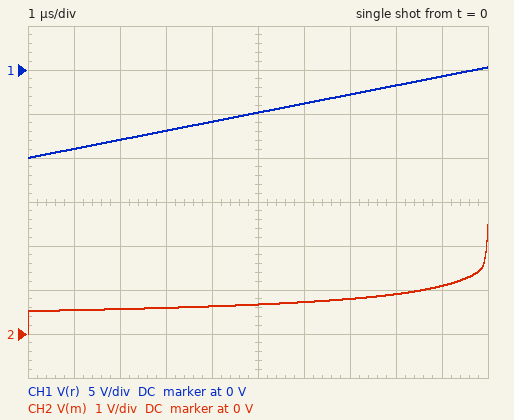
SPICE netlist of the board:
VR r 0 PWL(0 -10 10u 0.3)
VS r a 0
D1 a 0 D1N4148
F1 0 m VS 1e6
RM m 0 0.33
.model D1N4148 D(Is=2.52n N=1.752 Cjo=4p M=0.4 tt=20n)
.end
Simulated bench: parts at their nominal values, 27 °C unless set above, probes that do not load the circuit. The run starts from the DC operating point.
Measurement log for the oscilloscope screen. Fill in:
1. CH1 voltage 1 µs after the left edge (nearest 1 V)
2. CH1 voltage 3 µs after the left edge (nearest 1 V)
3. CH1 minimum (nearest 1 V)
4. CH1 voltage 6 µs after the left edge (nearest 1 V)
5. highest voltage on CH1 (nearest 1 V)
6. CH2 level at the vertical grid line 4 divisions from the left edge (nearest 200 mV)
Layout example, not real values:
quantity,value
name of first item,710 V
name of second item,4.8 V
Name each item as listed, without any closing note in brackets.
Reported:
quantity,value
CH1 voltage 1 µs after the left edge,-9 V
CH1 voltage 3 µs after the left edge,-7 V
CH1 minimum,-10 V
CH1 voltage 6 µs after the left edge,-4 V
highest voltage on CH1,0 V
CH2 level at the vertical grid line 4 divisions from the left edge,600 mV
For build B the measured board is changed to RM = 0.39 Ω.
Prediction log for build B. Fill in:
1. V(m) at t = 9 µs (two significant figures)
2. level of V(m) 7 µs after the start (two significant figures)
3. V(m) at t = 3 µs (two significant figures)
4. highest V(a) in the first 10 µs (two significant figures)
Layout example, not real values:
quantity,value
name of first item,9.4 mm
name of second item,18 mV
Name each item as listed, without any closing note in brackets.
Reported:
quantity,value
V(m) at t = 9 µs,1.3 V
level of V(m) 7 µs after the start,940 mV
V(m) at t = 3 µs,700 mV
highest V(a) in the first 10 µs,300 mV
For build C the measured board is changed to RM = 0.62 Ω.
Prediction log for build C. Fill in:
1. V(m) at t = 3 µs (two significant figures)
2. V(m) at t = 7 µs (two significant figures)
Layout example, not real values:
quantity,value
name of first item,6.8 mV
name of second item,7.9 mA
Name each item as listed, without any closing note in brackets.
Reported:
quantity,value
V(m) at t = 3 µs,1.1 V
V(m) at t = 7 µs,1.5 V
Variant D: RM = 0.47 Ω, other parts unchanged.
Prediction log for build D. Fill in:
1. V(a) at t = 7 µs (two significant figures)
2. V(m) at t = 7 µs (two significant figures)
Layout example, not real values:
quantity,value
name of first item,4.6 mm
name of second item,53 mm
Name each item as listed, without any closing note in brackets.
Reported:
quantity,value
V(a) at t = 7 µs,-2.8 V
V(m) at t = 7 µs,1.1 V
